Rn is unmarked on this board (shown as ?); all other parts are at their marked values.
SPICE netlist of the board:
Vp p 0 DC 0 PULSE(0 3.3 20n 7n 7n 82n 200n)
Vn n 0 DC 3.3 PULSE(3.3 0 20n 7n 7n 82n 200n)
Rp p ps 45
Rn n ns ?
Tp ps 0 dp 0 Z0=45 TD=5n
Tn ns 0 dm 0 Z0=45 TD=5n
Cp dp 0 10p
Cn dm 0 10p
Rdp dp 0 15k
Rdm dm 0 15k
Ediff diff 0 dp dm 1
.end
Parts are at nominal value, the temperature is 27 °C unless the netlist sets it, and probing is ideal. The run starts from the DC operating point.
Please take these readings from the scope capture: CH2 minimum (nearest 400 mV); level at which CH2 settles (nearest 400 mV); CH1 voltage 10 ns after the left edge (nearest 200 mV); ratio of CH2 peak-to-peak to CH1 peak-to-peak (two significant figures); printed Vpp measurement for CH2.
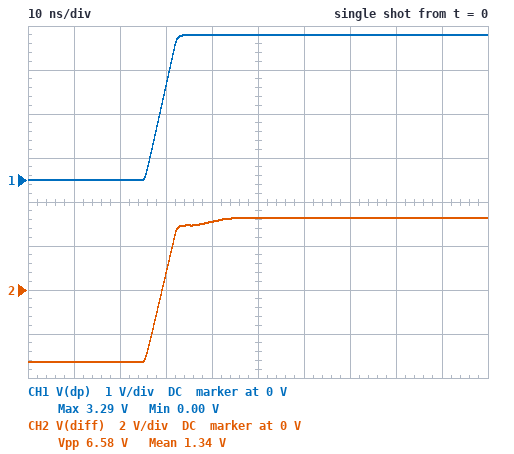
-3.2 V
3.2 V
0 V
2.0
6.58 V
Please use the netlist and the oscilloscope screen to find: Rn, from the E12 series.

56 Ω
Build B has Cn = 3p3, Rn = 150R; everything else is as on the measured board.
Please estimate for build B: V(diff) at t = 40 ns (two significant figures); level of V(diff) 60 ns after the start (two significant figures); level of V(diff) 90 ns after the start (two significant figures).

2.1 V
2.9 V
3.2 V
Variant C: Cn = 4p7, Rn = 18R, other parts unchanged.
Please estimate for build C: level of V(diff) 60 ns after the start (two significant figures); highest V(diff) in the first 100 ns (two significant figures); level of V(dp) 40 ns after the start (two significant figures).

3.4 V
4.7 V
3.3 V
